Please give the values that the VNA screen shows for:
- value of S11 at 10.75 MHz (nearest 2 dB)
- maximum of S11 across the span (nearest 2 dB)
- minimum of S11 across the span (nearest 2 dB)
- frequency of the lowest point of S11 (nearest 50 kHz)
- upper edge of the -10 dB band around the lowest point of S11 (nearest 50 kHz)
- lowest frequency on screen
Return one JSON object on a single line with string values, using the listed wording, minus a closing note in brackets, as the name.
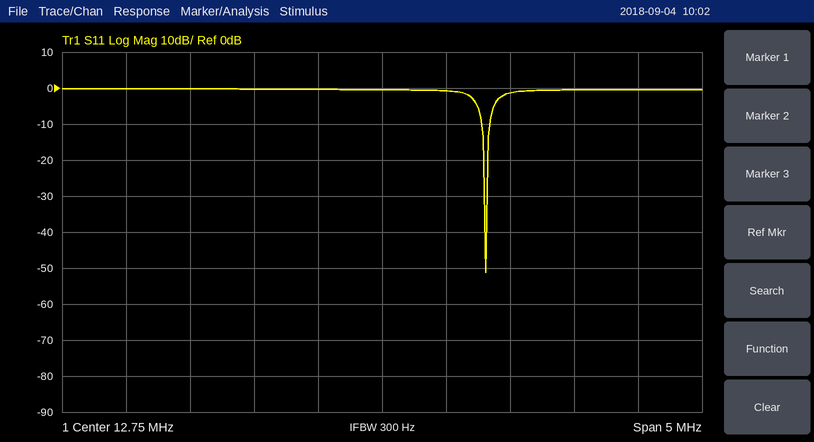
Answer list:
{"value of S11 at 10.75 MHz": "0 dB", "maximum of S11 across the span": "0 dB", "minimum of S11 across the span": "-52 dB", "frequency of the lowest point of S11": "13.55 MHz", "upper edge of the -10 dB band around the lowest point of S11": "13.60 MHz", "lowest frequency on screen": "10.25 MHz"}
